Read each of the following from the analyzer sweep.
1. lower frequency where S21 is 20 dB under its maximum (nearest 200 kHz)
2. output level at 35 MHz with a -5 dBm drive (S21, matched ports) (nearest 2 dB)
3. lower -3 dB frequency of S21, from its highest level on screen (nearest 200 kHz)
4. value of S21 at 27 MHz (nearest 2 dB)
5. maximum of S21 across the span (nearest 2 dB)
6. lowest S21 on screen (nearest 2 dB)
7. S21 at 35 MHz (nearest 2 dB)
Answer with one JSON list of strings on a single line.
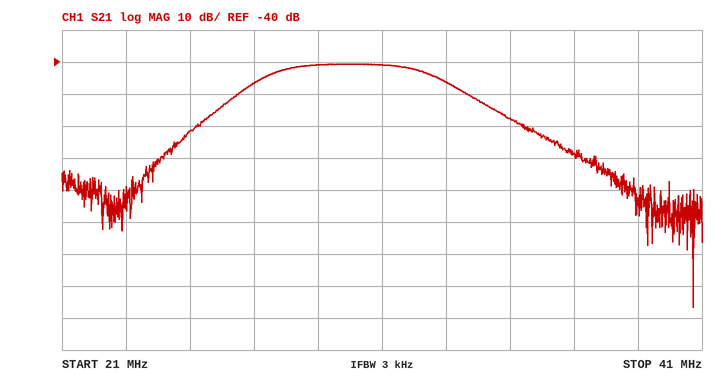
["25.2 MHz", "-62 dBm", "27.6 MHz", "-46 dB", "-40 dB", "-116 dB", "-58 dB"]
